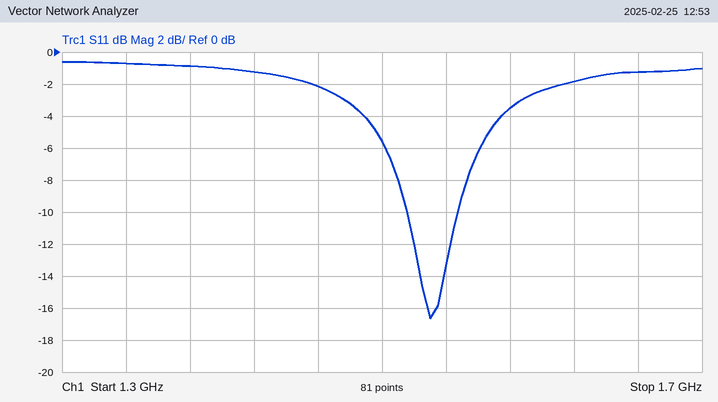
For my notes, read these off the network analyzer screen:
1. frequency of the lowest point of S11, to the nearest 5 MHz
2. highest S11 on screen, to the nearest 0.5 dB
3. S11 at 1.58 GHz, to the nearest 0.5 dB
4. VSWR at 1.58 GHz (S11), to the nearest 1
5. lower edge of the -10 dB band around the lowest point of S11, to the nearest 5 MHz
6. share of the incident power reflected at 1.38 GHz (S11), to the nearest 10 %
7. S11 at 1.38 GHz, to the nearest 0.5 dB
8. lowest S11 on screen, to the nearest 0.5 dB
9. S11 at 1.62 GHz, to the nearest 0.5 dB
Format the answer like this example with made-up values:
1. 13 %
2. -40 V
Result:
1. 1.530 GHz
2. -0.5 dB
3. -3.5 dB
4. 5
5. 1.515 GHz
6. 80 %
7. -1.0 dB
8. -16.5 dB
9. -2.0 dB
